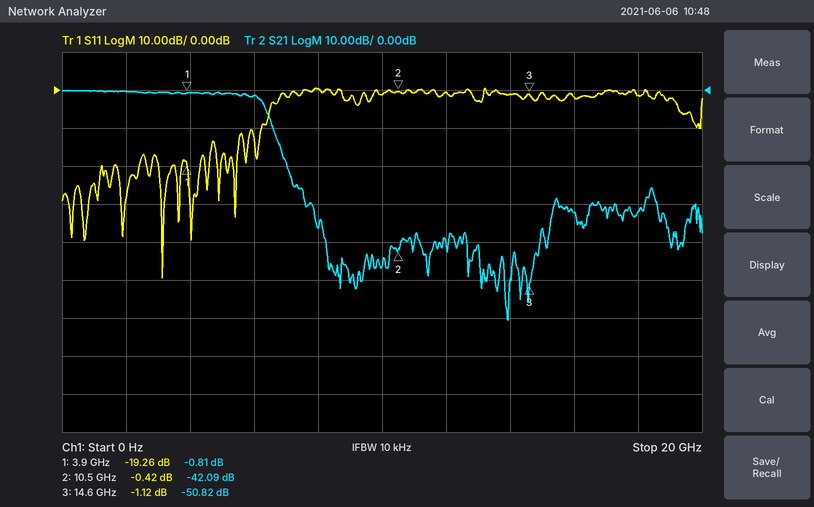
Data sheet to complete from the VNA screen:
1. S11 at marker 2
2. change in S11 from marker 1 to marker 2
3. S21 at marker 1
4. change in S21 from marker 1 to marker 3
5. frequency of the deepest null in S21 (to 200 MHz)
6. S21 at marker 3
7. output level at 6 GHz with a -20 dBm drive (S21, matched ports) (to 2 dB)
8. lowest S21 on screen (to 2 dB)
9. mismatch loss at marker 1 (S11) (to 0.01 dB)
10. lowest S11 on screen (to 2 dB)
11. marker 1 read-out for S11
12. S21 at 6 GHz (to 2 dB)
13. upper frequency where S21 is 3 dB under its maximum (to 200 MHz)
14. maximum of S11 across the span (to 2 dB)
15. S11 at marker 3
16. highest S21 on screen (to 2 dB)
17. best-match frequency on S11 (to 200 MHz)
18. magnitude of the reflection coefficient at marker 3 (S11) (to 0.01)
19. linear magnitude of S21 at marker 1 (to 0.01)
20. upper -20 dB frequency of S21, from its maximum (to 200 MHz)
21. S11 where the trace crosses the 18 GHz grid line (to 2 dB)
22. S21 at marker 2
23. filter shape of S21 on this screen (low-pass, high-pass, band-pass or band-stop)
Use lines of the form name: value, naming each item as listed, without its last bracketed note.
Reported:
S11 at marker 2: -0.42 dB
change in S11 from marker 1 to marker 2: 18.84 dB
S21 at marker 1: -0.81 dB
change in S21 from marker 1 to marker 3: -50.01 dB
frequency of the deepest null in S21: 14.0 GHz
S21 at marker 3: -50.82 dB
output level at 6 GHz with a -20 dBm drive (S21, matched ports): -22 dBm
lowest S21 on screen: -60 dB
mismatch loss at marker 1 (S11): 0.05 dB
lowest S11 on screen: -50 dB
marker 1 read-out for S11: -19.26 dB
S21 at 6 GHz: -2 dB
upper frequency where S21 is 3 dB under its maximum: 6.2 GHz
maximum of S11 across the span: 0 dB
S11 at marker 3: -1.12 dB
highest S21 on screen: 0 dB
best-match frequency on S11: 3.2 GHz
magnitude of the reflection coefficient at marker 3 (S11): 0.88
linear magnitude of S21 at marker 1: 0.91
upper -20 dB frequency of S21, from its maximum: 7.0 GHz
S11 where the trace crosses the 18 GHz grid line: -2 dB
S21 at marker 2: -42.09 dB
filter shape of S21 on this screen: low-pass
